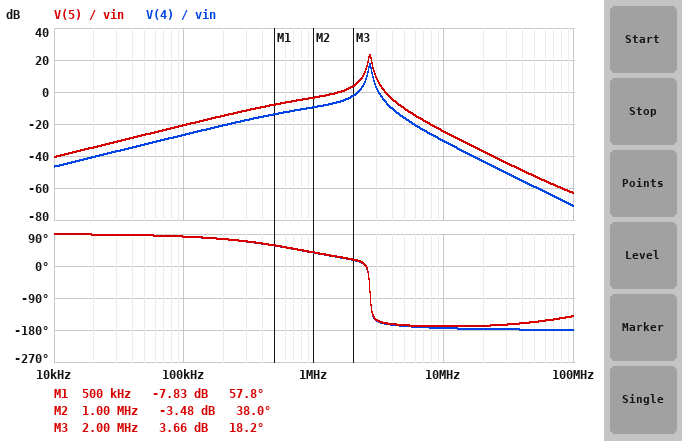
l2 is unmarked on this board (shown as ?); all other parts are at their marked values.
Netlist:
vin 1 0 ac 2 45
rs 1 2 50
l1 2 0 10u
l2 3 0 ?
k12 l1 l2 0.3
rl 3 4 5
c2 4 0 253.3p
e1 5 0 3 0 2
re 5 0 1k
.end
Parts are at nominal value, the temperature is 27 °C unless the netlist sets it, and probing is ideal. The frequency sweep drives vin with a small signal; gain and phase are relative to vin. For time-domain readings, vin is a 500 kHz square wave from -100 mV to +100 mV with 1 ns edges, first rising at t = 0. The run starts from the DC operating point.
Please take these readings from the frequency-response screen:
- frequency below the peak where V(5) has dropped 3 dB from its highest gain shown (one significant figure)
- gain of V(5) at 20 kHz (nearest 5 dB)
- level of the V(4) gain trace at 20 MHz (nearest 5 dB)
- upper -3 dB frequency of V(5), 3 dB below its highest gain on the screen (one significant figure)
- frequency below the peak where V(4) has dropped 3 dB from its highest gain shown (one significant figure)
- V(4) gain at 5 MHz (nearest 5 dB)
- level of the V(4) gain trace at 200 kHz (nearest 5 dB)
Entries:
3 MHz
-35 dB
-45 dB
3 MHz
3 MHz
-15 dB
-20 dB
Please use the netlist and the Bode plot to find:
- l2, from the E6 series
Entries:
15 µH
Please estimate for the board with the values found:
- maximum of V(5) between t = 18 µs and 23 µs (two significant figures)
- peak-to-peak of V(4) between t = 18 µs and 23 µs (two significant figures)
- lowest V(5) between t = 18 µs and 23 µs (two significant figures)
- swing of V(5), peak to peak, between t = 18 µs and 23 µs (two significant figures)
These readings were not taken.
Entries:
210 mV
210 mV
-210 mV
420 mV
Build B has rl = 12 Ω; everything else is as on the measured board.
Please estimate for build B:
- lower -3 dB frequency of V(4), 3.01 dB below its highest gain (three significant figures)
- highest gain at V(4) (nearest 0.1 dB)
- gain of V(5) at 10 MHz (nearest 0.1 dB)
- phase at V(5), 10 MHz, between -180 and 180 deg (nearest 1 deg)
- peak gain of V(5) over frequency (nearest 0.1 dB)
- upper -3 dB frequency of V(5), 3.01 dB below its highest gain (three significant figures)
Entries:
2.58 MHz
13.1 dB
-24.6 dB
-163 deg
19.1 dB
2.80 MHz
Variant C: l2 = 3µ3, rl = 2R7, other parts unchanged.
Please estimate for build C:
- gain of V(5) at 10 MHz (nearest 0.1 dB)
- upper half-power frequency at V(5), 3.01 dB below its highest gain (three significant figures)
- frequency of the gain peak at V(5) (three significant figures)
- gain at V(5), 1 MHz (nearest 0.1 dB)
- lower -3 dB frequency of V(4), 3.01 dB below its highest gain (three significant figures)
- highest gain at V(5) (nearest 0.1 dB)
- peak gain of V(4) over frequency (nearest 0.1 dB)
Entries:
-15.3 dB
5.87 MHz
5.76 MHz
-11.1 dB
5.65 MHz
19.0 dB
13.0 dB
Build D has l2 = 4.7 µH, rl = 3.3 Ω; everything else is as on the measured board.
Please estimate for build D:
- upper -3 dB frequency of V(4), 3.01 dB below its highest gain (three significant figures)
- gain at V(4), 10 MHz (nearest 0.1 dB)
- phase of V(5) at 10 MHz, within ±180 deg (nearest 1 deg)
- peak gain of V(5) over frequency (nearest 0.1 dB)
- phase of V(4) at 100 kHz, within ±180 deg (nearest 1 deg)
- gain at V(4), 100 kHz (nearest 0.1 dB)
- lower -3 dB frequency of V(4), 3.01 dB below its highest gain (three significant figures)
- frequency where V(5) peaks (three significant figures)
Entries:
4.93 MHz
-24.1 dB
-171 deg
19.9 dB
83 deg
-31.8 dB
4.73 MHz
4.83 MHz
